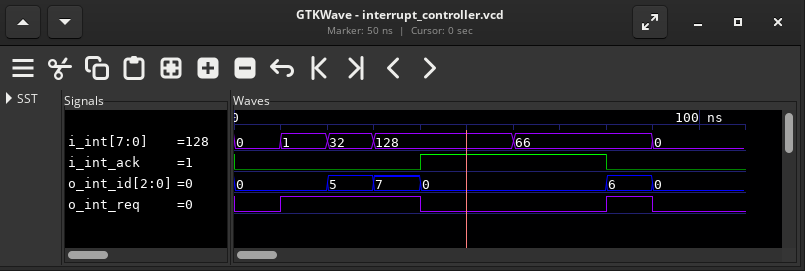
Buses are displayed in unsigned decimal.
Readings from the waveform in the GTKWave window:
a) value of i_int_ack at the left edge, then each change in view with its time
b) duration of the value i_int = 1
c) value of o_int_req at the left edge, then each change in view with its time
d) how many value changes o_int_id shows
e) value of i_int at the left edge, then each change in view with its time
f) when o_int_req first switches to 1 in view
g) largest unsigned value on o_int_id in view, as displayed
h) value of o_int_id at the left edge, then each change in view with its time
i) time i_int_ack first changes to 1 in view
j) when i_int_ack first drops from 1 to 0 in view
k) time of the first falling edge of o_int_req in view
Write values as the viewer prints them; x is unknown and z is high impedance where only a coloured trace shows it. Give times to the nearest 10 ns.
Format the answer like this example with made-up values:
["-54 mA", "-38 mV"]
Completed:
["0, 1 at 40 ns, 0 at 80 ns", "10 ns", "0, 1 at 10 ns, 0 at 40 ns, 1 at 80 ns, 0 at 90 ns", "5", "0, 1 at 10 ns, 32 at 20 ns, 128 at 30 ns, 66 at 60 ns, 0 at 90 ns", "10 ns", "7", "0, 5 at 20 ns, 7 at 30 ns, 0 at 40 ns, 6 at 80 ns, 0 at 90 ns", "40 ns", "80 ns", "40 ns"]
